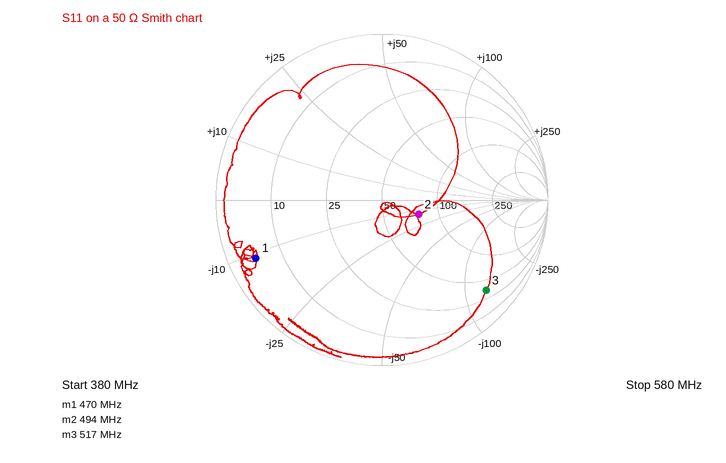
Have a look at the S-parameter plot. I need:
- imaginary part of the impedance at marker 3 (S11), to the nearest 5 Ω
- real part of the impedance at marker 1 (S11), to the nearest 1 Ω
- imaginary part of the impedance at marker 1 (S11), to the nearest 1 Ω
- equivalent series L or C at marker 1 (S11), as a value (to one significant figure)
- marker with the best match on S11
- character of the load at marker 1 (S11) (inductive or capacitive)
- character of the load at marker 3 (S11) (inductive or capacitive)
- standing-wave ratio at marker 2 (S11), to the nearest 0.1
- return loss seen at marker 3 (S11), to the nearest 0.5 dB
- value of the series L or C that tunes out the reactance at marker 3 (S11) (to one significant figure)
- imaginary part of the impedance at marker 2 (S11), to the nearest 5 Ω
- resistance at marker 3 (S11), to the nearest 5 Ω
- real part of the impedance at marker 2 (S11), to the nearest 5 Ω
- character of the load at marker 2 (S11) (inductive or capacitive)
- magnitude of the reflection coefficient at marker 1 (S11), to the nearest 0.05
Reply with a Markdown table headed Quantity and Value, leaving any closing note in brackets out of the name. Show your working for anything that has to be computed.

| Quantity | Value |
|---|---|
| imaginary part of the impedance at marker 3 (S11), to the nearest 5 Ω | -125 Ω |
| real part of the impedance at marker 1 (S11), to the nearest 1 Ω | 5 Ω |
| imaginary part of the impedance at marker 1 (S11), to the nearest 1 Ω | -11 Ω |
| equivalent series L or C at marker 1 (S11), as a value | C = 1/(2π × 470 MHz × 11 Ω) ≈ 30.8 pF, so 30 pF to one significant figure |
| marker with the best match on S11 | marker 2 |
| character of the load at marker 1 (S11) | capacitive |
| character of the load at marker 3 (S11) | capacitive |
| standing-wave ratio at marker 2 (S11), to the nearest 0.1 | 1.6 |
| return loss seen at marker 3 (S11), to the nearest 0.5 dB | 1.5 dB |
| value of the series L or C that tunes out the reactance at marker 3 (S11) | L = 125 Ω/(2π × 517 MHz) ≈ 38.5 nH, so 40 nH to one significant figure |
| imaginary part of the impedance at marker 2 (S11), to the nearest 5 Ω | -15 Ω |
| resistance at marker 3 (S11), to the nearest 5 Ω | 35 Ω |
| real part of the impedance at marker 2 (S11), to the nearest 5 Ω | 75 Ω |
| character of the load at marker 2 (S11) | capacitive |
| magnitude of the reflection coefficient at marker 1 (S11), to the nearest 0.05 | 0.85 |
